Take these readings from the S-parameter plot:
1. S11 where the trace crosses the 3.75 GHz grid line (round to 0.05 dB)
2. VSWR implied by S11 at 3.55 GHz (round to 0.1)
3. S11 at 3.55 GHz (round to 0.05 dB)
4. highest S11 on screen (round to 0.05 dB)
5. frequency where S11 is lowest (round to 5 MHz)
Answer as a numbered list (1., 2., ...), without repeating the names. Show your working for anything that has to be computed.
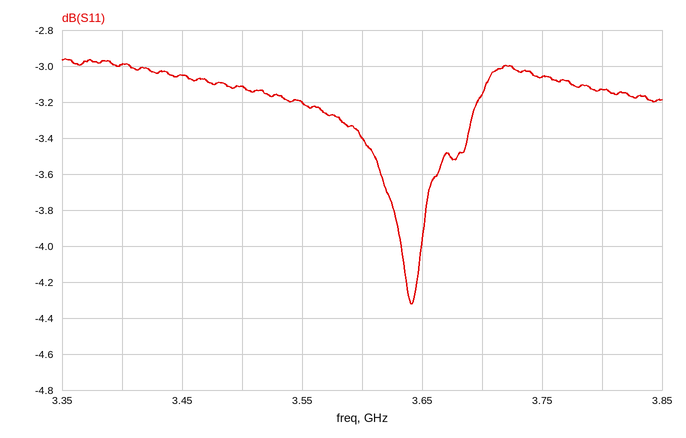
1. -3.05 dB
2. |Γ| = 10^(-3.2/20) = 0.6918; VSWR = (1 + 0.6918)/(1 − 0.6918) ≈ 5.5
3. -3.20 dB
4. -2.95 dB
5. 3.640 GHz
